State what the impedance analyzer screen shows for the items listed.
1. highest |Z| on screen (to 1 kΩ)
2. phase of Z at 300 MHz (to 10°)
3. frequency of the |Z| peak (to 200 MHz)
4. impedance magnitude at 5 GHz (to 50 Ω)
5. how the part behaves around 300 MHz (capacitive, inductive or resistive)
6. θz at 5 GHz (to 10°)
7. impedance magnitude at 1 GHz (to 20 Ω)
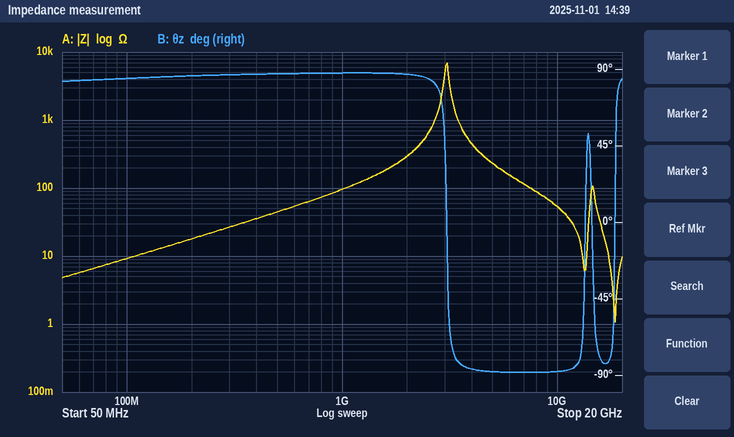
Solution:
7 kΩ
90°
3.0 GHz
250 Ω
inductive
-90°
100 Ω
